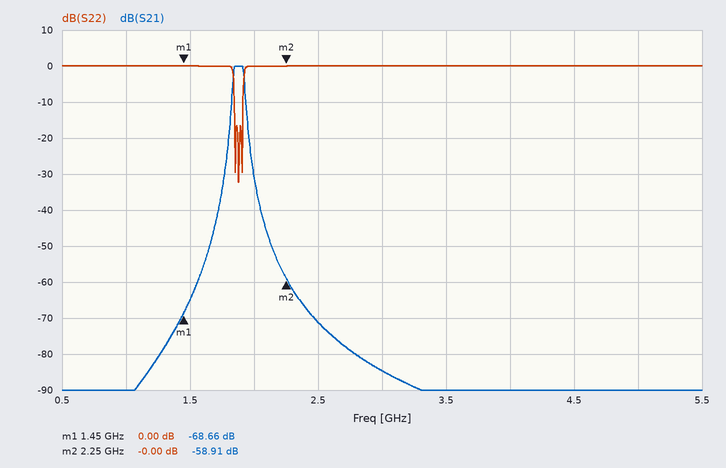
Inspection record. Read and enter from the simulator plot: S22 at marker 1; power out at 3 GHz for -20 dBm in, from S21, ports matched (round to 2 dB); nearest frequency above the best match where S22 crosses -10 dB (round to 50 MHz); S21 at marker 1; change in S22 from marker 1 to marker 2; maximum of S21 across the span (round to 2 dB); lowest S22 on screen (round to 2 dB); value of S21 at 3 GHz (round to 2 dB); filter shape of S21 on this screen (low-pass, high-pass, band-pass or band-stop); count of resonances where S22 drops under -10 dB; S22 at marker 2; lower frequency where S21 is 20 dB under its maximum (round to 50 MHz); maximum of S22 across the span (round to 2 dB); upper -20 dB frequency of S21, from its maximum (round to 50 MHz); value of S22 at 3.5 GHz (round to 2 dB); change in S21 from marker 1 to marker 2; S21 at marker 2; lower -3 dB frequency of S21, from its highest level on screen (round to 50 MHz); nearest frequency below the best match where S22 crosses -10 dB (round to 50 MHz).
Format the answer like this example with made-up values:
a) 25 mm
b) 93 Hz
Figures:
a) 0.00 dB
b) -104 dBm
c) 1.90 GHz
d) -68.66 dB
e) 0.00 dB
f) 0 dB
g) -32 dB
h) -84 dB
i) band-pass
j) 3
k) -0.00 dB
l) 1.80 GHz
m) 0 dB
n) 1.95 GHz
o) 0 dB
p) 9.75 dB
q) -58.91 dB
r) 1.85 GHz
s) 1.85 GHz
